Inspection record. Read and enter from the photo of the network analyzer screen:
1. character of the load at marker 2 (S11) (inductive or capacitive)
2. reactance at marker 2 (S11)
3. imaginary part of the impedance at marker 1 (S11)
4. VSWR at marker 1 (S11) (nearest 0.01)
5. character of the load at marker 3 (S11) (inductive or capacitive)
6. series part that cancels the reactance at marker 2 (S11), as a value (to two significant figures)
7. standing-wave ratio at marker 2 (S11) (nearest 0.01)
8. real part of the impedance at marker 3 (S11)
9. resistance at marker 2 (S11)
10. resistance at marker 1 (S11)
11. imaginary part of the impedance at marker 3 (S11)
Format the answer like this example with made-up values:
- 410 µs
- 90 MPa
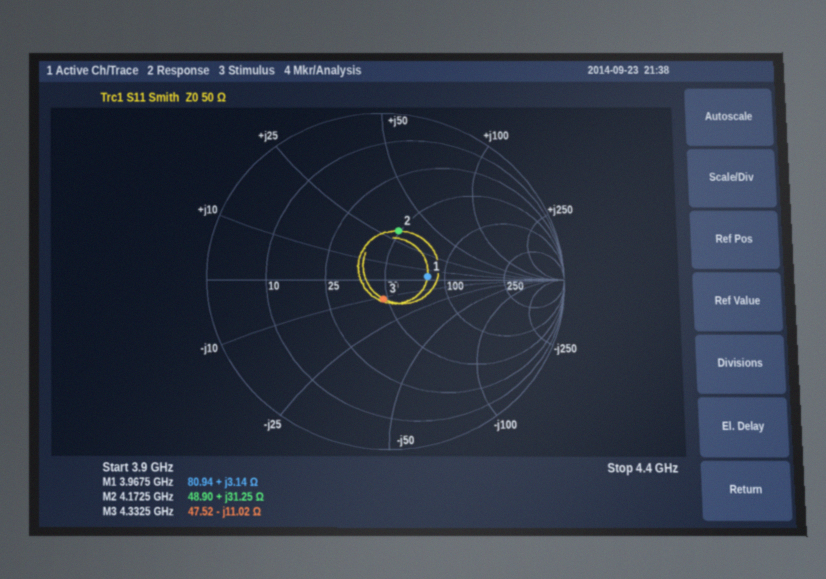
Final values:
- inductive
- +31.25 Ω
- +3.14 Ω
- 1.62
- capacitive
- 1.2 pF
- 1.86
- 47.52 Ω
- 48.90 Ω
- 80.94 Ω
- -11.02 Ω
